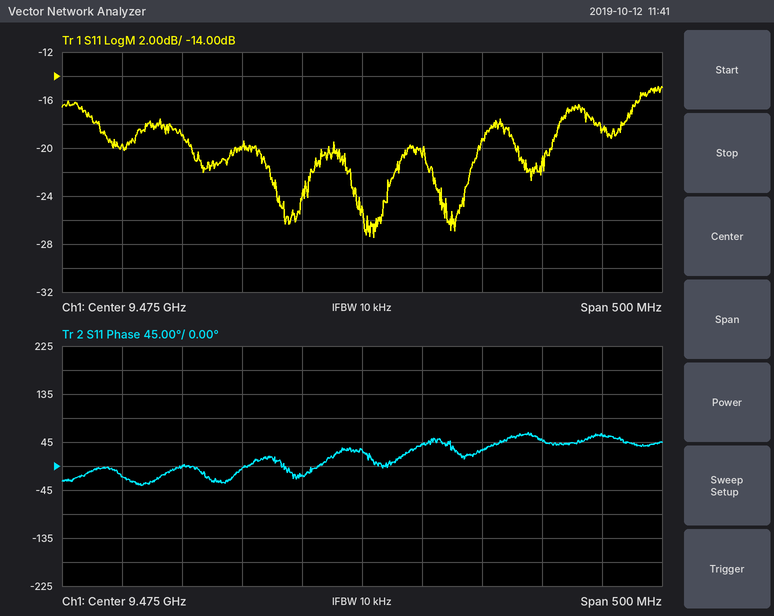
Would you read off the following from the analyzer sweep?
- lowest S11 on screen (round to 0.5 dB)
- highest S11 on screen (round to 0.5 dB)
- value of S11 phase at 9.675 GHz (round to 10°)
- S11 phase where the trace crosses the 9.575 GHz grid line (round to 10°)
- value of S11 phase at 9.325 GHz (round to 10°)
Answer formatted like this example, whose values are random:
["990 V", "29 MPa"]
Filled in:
["-27.5 dB", "-15.0 dB", "60°", "30°", "0°"]
